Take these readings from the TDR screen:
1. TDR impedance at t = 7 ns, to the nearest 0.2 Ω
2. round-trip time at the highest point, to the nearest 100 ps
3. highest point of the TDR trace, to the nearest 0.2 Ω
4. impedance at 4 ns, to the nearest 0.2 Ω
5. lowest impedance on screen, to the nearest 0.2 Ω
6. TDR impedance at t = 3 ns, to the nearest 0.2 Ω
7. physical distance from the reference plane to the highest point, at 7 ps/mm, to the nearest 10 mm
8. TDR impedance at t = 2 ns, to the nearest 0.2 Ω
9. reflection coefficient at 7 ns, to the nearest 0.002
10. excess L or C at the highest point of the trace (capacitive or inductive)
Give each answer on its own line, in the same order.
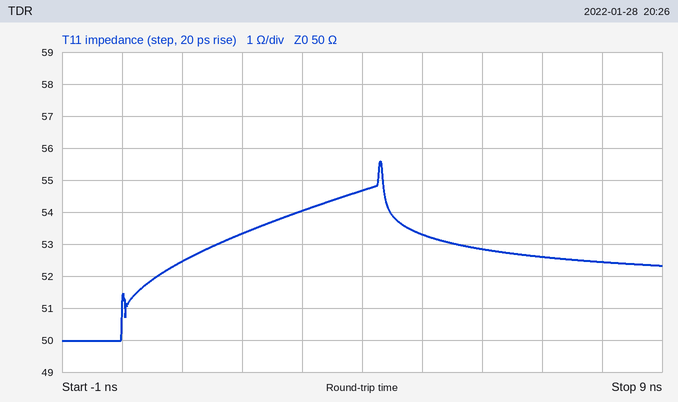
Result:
52.6 Ω
4.3 ns
55.6 Ω
54.6 Ω
50.0 Ω
54.0 Ω
310 mm
53.4 Ω
+0.026
inductive
